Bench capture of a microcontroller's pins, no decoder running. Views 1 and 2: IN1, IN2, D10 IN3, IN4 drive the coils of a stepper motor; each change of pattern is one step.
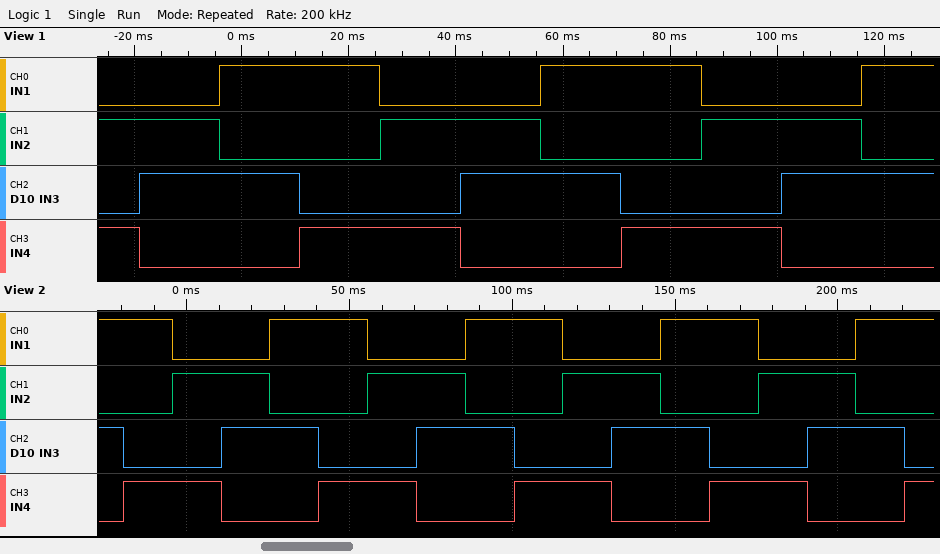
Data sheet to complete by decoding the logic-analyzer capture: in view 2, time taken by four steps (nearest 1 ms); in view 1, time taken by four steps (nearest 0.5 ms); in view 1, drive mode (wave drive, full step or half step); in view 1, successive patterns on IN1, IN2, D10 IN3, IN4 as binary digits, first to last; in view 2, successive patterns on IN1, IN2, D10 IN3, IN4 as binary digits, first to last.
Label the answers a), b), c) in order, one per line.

a) 60 ms
b) 60.0 ms
c) full step
d) 0101 0110 1010 1001 0101 0110 1010 1001 0101 0110 1010
e) 1010 1001 0101 0110 1010 1001 0101 0110 1010 1001 0101 0110 1010 1001 0101 0110 1010 1001
